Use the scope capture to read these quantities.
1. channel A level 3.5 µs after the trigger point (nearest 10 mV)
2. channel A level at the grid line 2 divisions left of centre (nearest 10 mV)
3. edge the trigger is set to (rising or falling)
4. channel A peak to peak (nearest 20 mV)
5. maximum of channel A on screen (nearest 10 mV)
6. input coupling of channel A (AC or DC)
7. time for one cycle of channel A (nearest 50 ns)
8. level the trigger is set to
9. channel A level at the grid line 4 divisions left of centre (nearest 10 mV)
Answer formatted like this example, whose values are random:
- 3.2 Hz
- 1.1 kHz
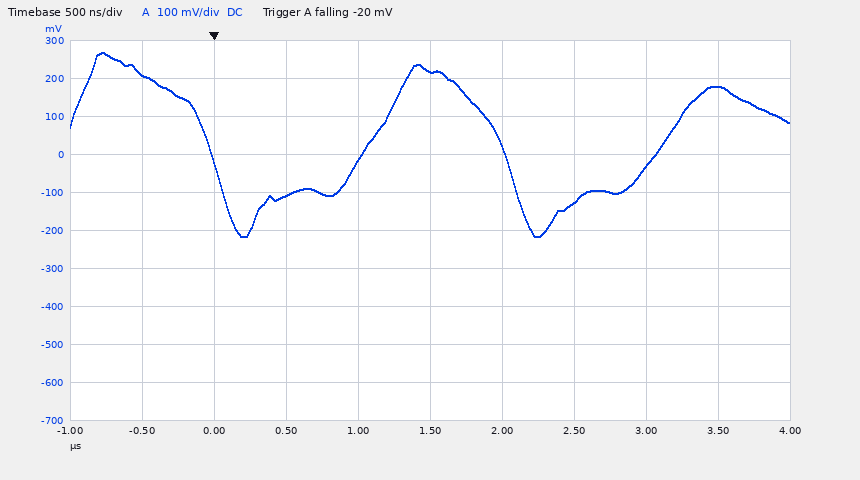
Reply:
- 180 mV
- -110 mV
- falling
- 480 mV
- 270 mV
- DC
- 2.05 µs
- -20 mV
- 210 mV
